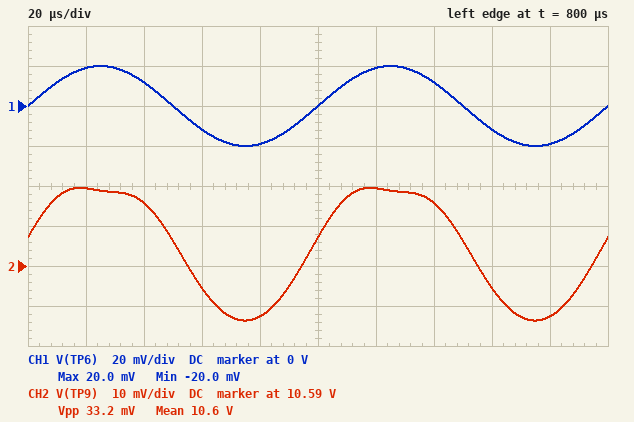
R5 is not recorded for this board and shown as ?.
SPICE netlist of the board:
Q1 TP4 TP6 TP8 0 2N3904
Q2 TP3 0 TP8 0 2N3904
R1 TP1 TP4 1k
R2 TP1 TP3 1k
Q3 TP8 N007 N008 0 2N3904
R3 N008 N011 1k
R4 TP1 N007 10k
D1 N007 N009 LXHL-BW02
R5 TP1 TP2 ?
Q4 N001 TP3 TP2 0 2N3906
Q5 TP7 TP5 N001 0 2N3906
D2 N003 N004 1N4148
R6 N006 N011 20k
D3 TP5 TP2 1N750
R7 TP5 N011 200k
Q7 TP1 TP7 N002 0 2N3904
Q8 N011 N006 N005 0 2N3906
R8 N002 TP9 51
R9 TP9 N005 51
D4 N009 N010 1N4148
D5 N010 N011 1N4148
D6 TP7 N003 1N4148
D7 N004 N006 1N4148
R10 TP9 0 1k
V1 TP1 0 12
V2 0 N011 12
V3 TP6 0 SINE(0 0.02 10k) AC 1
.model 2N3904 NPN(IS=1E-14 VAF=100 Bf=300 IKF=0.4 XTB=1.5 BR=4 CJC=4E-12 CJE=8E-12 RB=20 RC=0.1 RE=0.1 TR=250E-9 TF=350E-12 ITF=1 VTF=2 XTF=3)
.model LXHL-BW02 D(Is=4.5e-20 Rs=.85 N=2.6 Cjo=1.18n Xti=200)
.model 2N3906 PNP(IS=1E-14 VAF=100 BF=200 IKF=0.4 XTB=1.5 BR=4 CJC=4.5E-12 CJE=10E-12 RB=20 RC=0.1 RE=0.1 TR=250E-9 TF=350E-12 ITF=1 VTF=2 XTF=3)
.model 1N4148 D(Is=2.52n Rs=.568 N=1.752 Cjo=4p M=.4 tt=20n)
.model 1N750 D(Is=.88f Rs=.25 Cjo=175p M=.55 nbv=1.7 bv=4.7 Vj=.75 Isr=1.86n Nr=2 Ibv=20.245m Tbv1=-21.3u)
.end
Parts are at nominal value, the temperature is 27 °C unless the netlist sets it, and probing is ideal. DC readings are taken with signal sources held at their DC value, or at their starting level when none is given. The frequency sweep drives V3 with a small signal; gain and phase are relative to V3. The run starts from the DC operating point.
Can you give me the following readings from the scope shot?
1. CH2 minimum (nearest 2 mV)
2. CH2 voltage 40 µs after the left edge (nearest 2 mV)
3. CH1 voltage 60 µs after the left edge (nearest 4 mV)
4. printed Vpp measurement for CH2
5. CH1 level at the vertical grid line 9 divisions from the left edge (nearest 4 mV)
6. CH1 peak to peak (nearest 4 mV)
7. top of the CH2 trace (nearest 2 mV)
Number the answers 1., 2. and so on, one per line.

1. 10.576 V
2. 10.606 V
3. -12 mV
4. 33.2 mV
5. -20 mV
6. 40 mV
7. 10.610 V
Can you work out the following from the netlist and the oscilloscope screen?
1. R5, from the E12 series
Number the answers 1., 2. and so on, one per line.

1. 47 Ω
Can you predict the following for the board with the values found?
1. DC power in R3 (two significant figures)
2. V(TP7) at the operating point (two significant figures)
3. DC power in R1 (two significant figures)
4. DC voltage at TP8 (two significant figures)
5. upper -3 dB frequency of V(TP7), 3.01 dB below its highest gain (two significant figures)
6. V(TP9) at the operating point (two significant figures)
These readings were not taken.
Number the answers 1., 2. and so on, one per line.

1. 9.8 mW
2. 12 V
3. 2.4 mW
4. -660 mV
5. 62 MHz
6. 11 V
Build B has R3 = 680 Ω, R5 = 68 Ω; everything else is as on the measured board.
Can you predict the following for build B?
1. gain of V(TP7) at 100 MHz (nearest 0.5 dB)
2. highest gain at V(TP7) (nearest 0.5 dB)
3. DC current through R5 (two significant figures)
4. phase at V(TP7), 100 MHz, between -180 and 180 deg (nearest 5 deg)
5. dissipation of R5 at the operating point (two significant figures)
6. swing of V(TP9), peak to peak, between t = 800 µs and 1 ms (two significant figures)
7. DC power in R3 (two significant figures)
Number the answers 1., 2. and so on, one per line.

1. 3.0 dB
2. 9.0 dB
3. 2.6 mA
4. -55 deg
5. 470 µW
6. 90 mV
7. 14 mW
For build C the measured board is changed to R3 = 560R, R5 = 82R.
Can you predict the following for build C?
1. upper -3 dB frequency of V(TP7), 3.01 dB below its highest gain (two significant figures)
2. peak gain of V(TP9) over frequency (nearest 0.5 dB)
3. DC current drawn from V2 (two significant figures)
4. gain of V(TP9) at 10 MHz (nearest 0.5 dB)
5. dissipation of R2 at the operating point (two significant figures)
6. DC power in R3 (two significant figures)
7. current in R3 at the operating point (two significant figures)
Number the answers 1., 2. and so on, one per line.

1. 42 MHz
2. 11.5 dB
3. 8.8 mA
4. 11.0 dB
5. 1.0 mW
6. 17 mW
7. 5.6 mA
